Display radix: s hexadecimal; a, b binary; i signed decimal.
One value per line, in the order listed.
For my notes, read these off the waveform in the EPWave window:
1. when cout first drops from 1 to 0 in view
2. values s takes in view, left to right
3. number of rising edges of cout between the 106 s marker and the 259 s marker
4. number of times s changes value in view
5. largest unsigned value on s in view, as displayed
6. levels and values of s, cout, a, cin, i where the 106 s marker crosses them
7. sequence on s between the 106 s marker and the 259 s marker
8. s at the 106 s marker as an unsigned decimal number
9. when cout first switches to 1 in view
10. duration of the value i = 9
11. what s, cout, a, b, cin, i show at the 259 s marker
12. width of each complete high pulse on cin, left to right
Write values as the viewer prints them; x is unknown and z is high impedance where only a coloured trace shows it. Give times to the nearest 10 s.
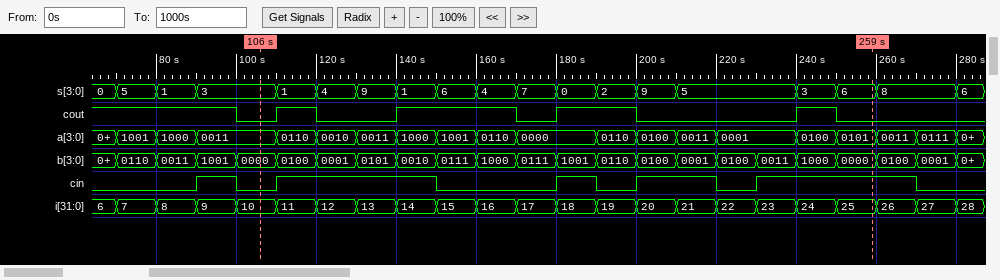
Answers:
100 s
0, 5, 1, 3, 1, 4, 9, 1, 6, 4, 7, 0, 2, 9, 5, 3, 6, 8, 6
4
18
9
s=3, cout=0, a=0011, cin=0, i=10
3, 1, 4, 9, 1, 6, 4, 7, 0, 2, 9, 5, 3, 6
3
110 s
10 s
s=6, cout=0, a=0101, b=0000, cin=1, i=25
10 s, 40 s, 10 s, 20 s, 40 s
